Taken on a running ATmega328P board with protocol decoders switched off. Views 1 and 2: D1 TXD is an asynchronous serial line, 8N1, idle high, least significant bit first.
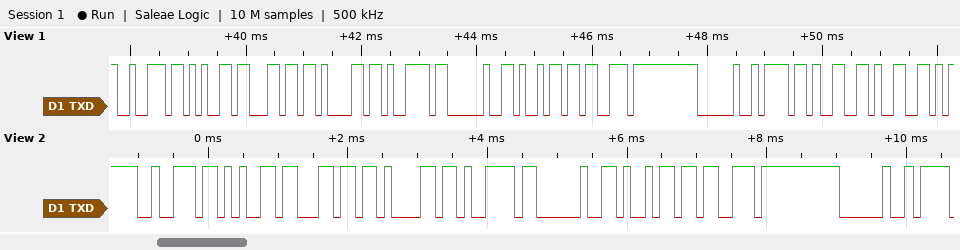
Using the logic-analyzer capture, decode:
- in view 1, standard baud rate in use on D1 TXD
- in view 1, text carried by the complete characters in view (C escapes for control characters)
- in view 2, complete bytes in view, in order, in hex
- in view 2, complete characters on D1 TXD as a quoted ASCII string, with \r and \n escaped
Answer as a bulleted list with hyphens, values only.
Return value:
- 9600 baud
- "relay is off"
- 72 65 6C 61 79 20 69 73 20
- "relay is "
